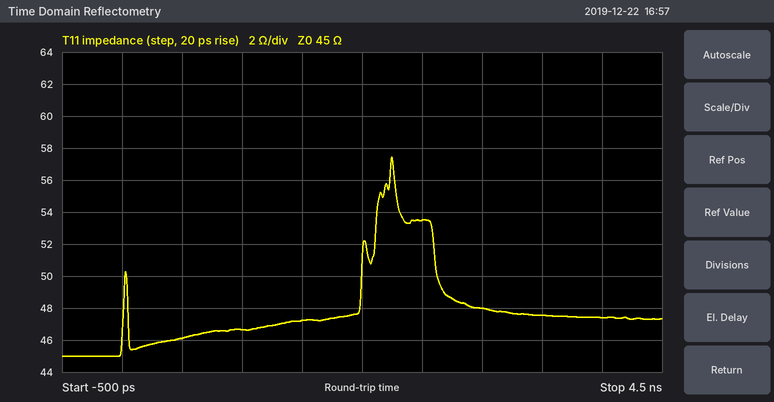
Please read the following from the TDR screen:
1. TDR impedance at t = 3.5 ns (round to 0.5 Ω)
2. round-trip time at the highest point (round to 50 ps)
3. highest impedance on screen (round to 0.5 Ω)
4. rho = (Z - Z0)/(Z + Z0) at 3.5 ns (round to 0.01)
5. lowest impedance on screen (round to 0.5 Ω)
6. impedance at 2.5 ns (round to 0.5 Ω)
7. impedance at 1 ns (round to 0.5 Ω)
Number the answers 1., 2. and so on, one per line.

1. 47.5 Ω
2. 2.25 ns
3. 57.5 Ω
4. +0.03
5. 45.0 Ω
6. 53.5 Ω
7. 46.5 Ω
